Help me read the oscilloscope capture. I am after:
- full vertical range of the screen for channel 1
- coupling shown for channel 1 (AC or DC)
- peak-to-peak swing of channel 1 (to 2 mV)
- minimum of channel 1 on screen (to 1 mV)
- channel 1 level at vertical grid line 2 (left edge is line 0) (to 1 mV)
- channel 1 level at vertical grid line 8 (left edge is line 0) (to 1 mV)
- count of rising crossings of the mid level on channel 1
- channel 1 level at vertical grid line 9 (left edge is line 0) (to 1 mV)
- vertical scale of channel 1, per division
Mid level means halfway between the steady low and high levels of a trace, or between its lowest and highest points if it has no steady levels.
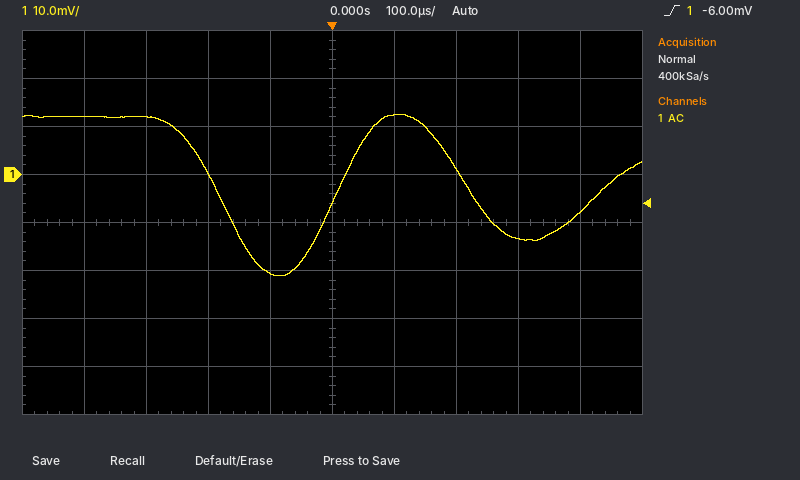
80 mV
AC
34 mV
-21 mV
12 mV
-13 mV
2
-8 mV
10 mV
